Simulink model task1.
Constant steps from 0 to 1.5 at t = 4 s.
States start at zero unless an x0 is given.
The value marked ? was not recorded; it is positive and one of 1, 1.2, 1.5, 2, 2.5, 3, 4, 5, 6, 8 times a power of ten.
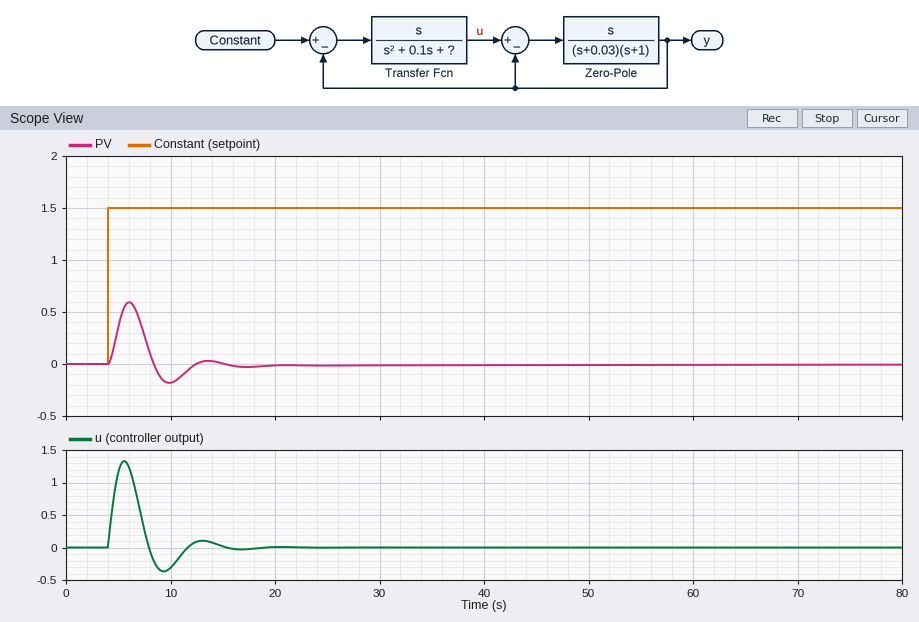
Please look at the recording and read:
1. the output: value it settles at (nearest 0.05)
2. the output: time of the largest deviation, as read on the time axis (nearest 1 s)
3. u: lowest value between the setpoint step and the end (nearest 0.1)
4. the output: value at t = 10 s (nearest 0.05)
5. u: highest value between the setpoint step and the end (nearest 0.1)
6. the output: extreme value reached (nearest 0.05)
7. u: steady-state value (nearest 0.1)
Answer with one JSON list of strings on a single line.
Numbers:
["0.00", "6 s", "-0.4", "-0.20", "1.3", "0.60", "0.0"]
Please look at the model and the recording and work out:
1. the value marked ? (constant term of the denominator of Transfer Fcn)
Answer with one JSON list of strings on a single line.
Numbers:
["0.6"]
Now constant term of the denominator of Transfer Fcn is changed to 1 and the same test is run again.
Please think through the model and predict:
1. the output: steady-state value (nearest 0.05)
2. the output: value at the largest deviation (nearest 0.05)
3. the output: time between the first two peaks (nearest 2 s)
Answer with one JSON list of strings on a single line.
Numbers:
["0.00", "0.50", "6 s"]
